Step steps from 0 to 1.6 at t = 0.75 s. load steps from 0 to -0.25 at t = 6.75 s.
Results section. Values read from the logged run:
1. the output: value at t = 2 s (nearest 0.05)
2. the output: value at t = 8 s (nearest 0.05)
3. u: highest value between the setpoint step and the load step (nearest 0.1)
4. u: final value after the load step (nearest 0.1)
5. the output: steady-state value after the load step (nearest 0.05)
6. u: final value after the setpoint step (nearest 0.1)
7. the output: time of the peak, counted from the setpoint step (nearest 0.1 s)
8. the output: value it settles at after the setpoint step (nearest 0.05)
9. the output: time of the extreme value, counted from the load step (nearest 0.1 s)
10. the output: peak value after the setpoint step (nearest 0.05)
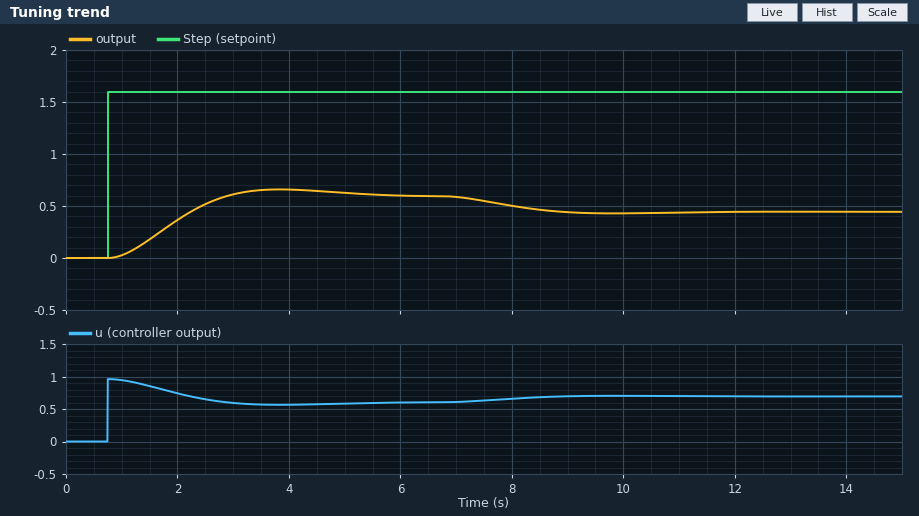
0.35
0.50
1.0
0.7
0.45
0.6
3.1 s
0.60
3.1 s
0.65
